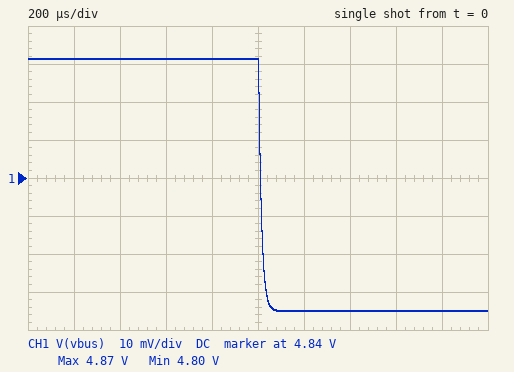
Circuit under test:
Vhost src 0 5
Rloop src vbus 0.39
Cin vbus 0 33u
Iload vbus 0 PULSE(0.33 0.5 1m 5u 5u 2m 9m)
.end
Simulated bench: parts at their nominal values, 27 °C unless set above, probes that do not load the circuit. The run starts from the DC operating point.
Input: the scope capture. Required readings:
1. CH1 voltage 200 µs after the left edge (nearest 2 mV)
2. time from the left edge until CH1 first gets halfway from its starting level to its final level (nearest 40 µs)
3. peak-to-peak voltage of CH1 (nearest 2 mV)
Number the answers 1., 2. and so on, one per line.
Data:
1. 4.872 V
2. 1.00 ms
3. 66 mV
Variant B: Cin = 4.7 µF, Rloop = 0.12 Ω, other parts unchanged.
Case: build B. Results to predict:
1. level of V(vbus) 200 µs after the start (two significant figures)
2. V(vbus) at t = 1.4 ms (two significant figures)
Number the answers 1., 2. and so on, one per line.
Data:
1. 5.0 V
2. 4.9 V
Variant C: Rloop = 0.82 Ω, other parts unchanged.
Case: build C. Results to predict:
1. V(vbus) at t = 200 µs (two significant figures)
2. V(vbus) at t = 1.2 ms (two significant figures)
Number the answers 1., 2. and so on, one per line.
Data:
1. 4.7 V
2. 4.6 V
